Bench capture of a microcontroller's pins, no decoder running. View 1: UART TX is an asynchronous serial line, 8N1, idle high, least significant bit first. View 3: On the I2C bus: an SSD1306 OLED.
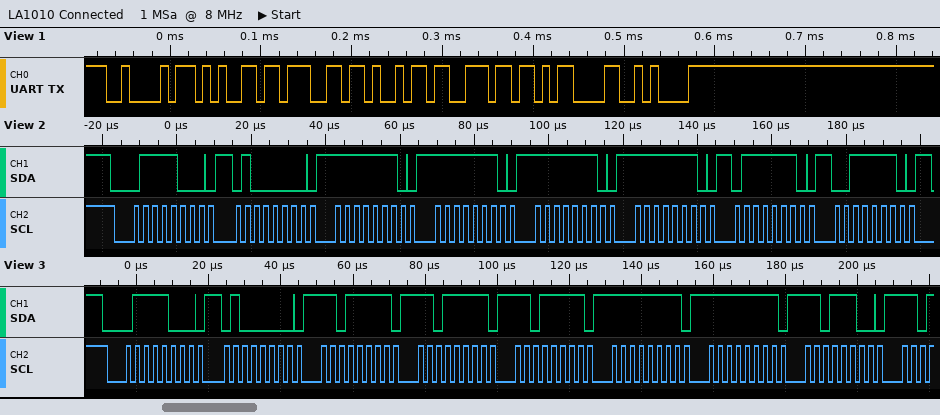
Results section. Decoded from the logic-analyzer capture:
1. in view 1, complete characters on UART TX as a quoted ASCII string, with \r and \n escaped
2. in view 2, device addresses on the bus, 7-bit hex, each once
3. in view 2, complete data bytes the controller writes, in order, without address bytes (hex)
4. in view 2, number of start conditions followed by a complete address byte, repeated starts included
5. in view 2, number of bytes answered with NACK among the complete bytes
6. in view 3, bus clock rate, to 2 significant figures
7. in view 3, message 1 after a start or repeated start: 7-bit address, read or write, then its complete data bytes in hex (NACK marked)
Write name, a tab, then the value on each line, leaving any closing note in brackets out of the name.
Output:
in view 1, complete characters on UART TX as a quoted ASCII string, with \r and \n escaped	"Begin\r\n"
in view 2, device addresses on the bus, 7-bit hex, each once	0x3C
in view 2, complete data bytes the controller writes, in order, without address bytes	40 FE FE FE FE 7E 3E
in view 2, number of start conditions followed by a complete address byte, repeated starts included	1
in view 2, number of bytes answered with NACK among the complete bytes	0
in view 3, bus clock rate, to 2 significant figures	400 kHz
in view 3, message 1 after a start or repeated start: 7-bit address, read or write, then its complete data bytes in hex	0x3C write: 40 DF DF DF FF FF DC
